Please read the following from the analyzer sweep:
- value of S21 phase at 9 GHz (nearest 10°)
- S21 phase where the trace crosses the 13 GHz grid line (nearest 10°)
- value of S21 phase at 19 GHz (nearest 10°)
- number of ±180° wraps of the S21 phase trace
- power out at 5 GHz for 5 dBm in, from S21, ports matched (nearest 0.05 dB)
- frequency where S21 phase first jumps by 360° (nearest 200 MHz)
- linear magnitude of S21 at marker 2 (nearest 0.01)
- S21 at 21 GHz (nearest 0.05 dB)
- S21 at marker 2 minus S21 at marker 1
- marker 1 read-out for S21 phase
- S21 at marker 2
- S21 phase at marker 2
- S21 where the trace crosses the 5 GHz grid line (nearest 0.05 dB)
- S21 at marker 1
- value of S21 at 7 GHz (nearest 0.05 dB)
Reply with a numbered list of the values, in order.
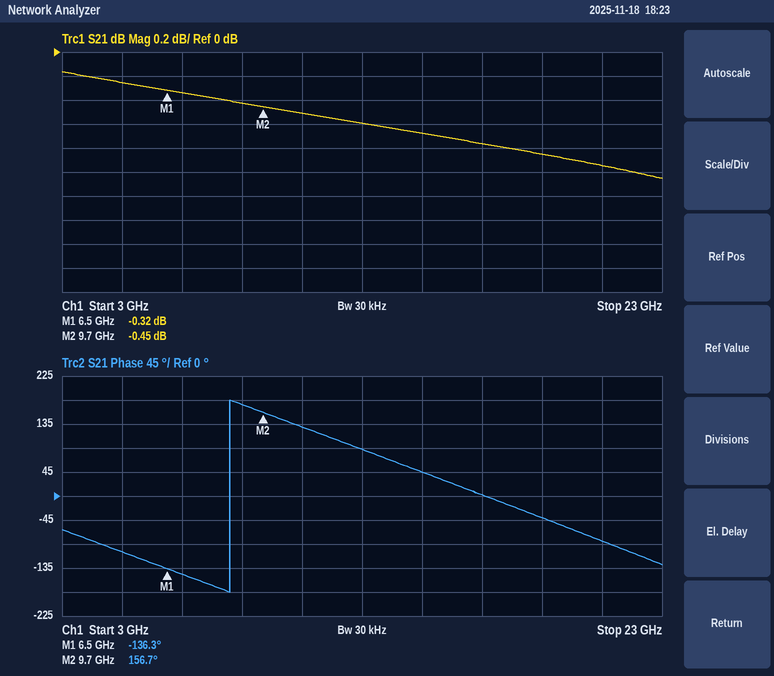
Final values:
1. 170°
2. 90°
3. -40°
4. 1
5. 4.75 dBm
6. 8.6 GHz
7. 0.95
8. -0.95 dB
9. -0.13 dB
10. -136.3°
11. -0.45 dB
12. 156.7°
13. -0.25 dB
14. -0.32 dB
15. -0.35 dB
